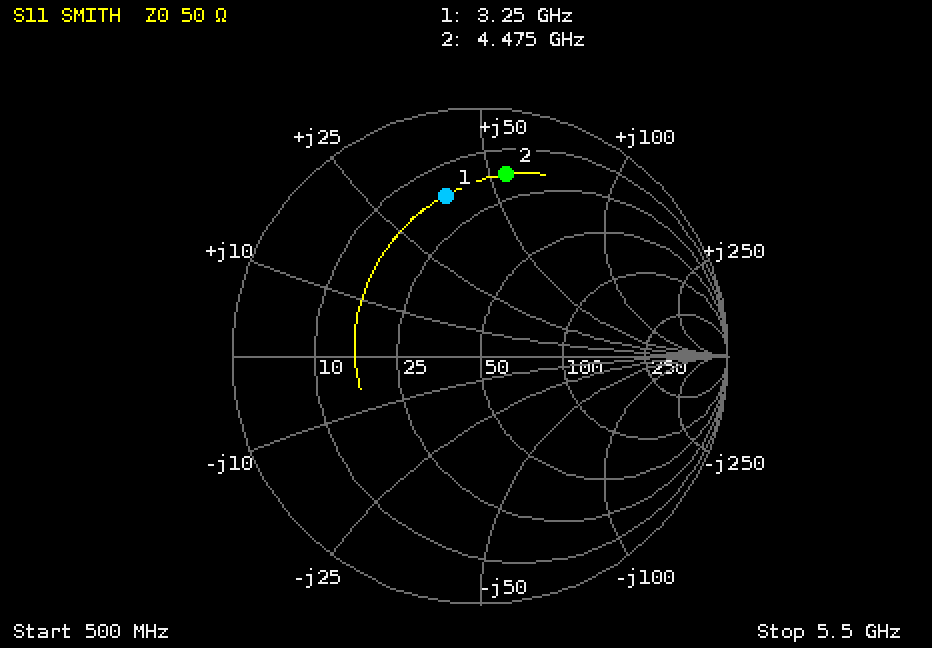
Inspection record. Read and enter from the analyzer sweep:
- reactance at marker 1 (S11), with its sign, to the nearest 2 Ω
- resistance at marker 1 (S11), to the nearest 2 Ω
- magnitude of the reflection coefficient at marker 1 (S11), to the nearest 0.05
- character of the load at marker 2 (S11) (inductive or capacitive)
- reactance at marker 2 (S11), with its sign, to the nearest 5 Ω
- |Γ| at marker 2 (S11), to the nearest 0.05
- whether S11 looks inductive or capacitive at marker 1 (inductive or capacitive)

+38 Ω
16 Ω
0.65
inductive
+55 Ω
0.75
inductive
